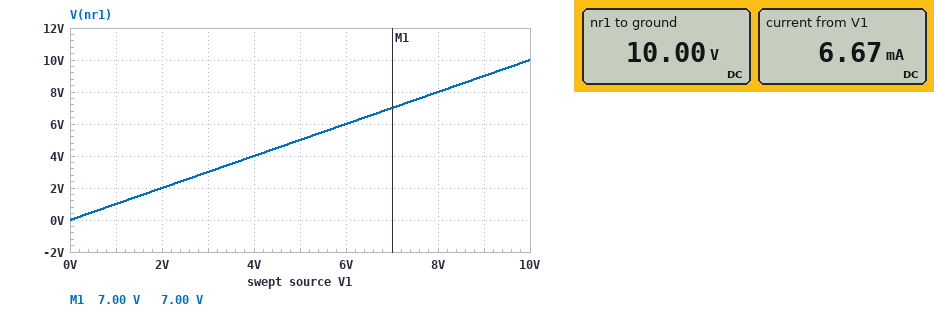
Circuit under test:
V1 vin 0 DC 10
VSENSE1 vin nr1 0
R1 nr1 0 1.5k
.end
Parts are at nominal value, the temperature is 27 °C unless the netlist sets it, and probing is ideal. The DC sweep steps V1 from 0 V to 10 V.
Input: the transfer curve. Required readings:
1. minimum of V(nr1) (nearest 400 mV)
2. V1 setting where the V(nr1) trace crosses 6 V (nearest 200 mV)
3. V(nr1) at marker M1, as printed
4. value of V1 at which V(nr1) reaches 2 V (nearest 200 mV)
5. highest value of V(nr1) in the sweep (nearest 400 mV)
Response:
0 V
6.0 V
7.00 V
2.0 V
10.0 V
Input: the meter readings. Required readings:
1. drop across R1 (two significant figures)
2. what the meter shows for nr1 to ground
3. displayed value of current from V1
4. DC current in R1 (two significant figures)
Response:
10 V
10.00 V
6.67 mA
6.7 mA
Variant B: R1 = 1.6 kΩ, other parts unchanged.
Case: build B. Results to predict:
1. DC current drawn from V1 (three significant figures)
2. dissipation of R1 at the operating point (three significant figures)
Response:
6.25 mA
62.5 mW
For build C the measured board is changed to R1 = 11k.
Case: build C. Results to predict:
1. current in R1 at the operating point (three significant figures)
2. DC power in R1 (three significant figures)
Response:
909 µA
9.09 mW
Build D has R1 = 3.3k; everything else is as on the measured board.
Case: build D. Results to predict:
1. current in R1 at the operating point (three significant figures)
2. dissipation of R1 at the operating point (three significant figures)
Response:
3.03 mA
30.3 mW
